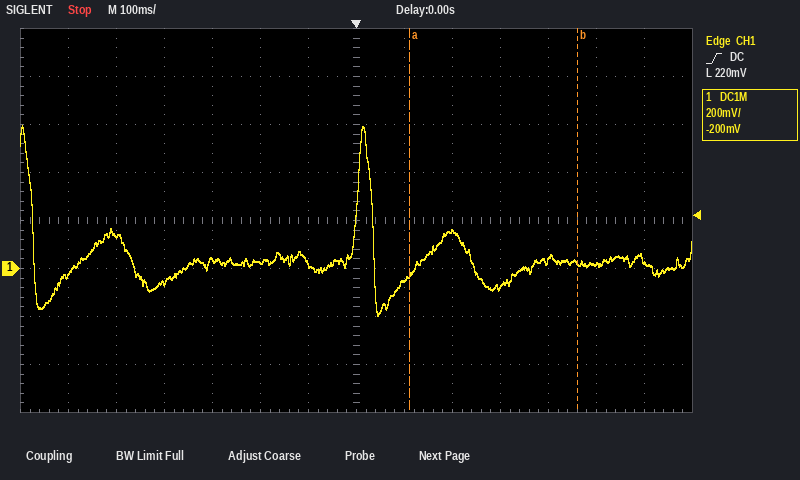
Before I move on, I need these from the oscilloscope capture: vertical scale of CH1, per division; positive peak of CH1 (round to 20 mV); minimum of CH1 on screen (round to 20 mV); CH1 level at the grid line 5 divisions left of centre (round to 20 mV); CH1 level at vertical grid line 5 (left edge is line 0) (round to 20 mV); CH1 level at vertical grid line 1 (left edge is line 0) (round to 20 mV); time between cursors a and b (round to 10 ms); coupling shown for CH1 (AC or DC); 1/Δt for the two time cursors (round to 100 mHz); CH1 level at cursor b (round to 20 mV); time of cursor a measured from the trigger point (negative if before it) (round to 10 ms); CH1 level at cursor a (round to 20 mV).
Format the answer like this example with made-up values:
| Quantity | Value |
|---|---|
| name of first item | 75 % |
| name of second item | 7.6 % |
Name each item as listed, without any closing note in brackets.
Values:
| Quantity | Value |
|---|---|
| vertical scale of CH1, per division | 200 mV |
| positive peak of CH1 | 600 mV |
| minimum of CH1 on screen | -200 mV |
| CH1 level at the grid line 5 divisions left of centre | 140 mV |
| CH1 level at vertical grid line 5 (left edge is line 0) | 20 mV |
| CH1 level at vertical grid line 1 (left edge is line 0) | -20 mV |
| time between cursors a and b | 350 ms |
| coupling shown for CH1 | DC |
| 1/Δt for the two time cursors | 2.9 Hz |
| CH1 level at cursor b | 20 mV |
| time of cursor a measured from the trigger point (negative if before it) | +110 ms |
| CH1 level at cursor a | -20 mV |
